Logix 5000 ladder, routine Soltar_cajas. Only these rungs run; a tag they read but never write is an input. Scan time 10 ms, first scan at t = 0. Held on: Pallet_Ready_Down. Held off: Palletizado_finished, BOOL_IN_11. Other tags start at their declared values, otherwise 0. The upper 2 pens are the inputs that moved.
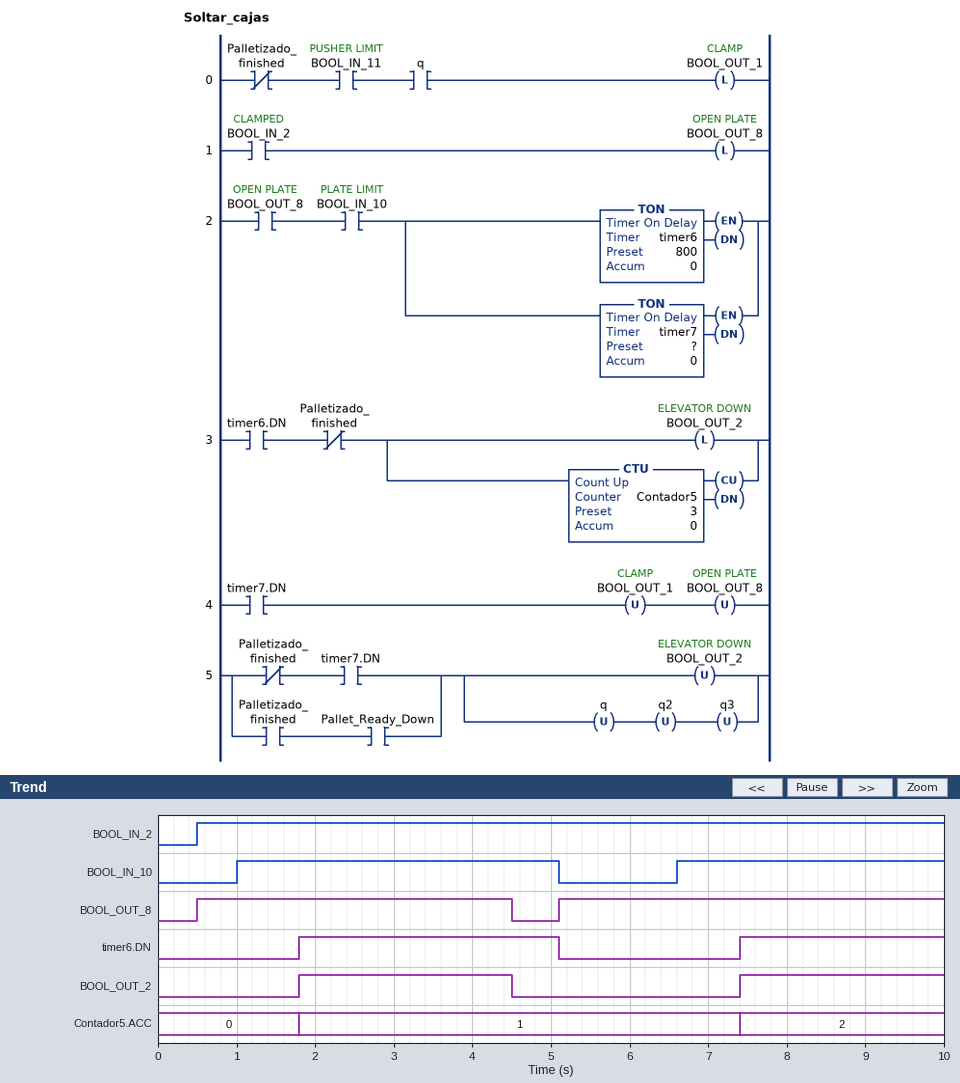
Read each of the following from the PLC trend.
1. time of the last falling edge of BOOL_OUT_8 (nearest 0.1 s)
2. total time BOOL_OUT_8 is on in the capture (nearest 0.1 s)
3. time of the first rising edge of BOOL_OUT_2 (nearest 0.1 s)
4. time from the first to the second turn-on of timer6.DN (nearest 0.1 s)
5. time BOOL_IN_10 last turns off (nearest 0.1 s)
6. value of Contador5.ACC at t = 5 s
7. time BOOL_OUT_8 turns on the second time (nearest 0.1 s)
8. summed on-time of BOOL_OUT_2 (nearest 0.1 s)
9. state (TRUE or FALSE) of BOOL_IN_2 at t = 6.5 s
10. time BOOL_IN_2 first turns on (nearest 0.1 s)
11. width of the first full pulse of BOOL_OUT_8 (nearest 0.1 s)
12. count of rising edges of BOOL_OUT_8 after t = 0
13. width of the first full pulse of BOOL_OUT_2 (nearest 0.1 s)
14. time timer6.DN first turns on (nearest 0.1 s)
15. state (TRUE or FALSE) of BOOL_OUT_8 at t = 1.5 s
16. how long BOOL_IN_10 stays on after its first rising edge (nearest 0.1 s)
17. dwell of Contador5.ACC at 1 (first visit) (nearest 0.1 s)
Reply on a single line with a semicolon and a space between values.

4.5 s; 8.9 s; 1.8 s; 5.6 s; 5.1 s; 1; 5.1 s; 5.3 s; TRUE; 0.5 s; 4.0 s; 2; 2.7 s; 1.8 s; TRUE; 4.1 s; 5.6 s
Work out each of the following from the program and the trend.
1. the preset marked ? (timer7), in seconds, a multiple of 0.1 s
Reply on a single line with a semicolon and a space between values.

3.5 s
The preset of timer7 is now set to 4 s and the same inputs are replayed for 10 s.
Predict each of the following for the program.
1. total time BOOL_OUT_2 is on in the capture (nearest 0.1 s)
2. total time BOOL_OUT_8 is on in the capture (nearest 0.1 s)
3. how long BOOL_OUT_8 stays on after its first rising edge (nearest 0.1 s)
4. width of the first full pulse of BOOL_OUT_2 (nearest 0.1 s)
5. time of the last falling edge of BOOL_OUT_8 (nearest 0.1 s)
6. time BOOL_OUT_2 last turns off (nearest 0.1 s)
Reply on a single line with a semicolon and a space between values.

5.8 s; 9.4 s; 4.5 s; 3.2 s; 5.0 s; 5.0 s
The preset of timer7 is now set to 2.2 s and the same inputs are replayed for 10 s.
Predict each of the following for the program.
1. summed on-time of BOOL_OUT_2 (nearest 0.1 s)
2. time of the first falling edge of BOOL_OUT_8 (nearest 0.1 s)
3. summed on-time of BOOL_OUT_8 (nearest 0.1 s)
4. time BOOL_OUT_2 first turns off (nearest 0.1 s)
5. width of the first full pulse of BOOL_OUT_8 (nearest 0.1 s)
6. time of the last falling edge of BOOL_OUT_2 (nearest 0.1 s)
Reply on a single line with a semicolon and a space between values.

2.8 s; 3.2 s; 6.4 s; 3.2 s; 2.7 s; 8.8 s
